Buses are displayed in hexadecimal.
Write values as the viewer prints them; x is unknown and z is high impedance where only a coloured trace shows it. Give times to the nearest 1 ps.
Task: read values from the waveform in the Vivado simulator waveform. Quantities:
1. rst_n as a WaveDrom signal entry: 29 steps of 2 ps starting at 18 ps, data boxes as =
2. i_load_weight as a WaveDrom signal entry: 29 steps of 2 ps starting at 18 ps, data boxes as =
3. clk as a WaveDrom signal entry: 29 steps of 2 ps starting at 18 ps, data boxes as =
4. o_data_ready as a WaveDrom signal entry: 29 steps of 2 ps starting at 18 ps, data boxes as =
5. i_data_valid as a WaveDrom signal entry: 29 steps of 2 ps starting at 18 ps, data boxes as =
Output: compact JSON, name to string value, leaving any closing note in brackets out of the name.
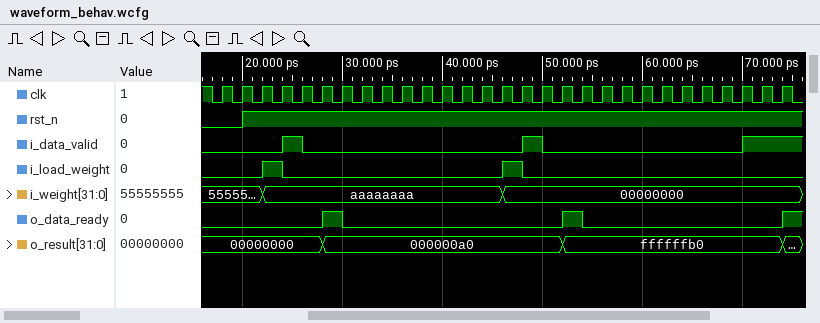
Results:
{"rst_n as a WaveDrom signal entry: 29 steps of 2 ps starting at 18 ps, data boxes as =": "{name: 'rst_n', wave: '01...........................'}", "i_load_weight as a WaveDrom signal entry: 29 steps of 2 ps starting at 18 ps, data boxes as =": "{name: 'i_load_weight', wave: '0.10..........10.............'}", "clk as a WaveDrom signal entry: 29 steps of 2 ps starting at 18 ps, data boxes as =": "{name: 'clk', wave: 'p............................'}", "o_data_ready as a WaveDrom signal entry: 29 steps of 2 ps starting at 18 ps, data boxes as =": "{name: 'o_data_ready', wave: '0....10..........10.........1'}", "i_data_valid as a WaveDrom signal entry: 29 steps of 2 ps starting at 18 ps, data boxes as =": "{name: 'i_data_valid', wave: '0..10..........10.........1..'}"}
